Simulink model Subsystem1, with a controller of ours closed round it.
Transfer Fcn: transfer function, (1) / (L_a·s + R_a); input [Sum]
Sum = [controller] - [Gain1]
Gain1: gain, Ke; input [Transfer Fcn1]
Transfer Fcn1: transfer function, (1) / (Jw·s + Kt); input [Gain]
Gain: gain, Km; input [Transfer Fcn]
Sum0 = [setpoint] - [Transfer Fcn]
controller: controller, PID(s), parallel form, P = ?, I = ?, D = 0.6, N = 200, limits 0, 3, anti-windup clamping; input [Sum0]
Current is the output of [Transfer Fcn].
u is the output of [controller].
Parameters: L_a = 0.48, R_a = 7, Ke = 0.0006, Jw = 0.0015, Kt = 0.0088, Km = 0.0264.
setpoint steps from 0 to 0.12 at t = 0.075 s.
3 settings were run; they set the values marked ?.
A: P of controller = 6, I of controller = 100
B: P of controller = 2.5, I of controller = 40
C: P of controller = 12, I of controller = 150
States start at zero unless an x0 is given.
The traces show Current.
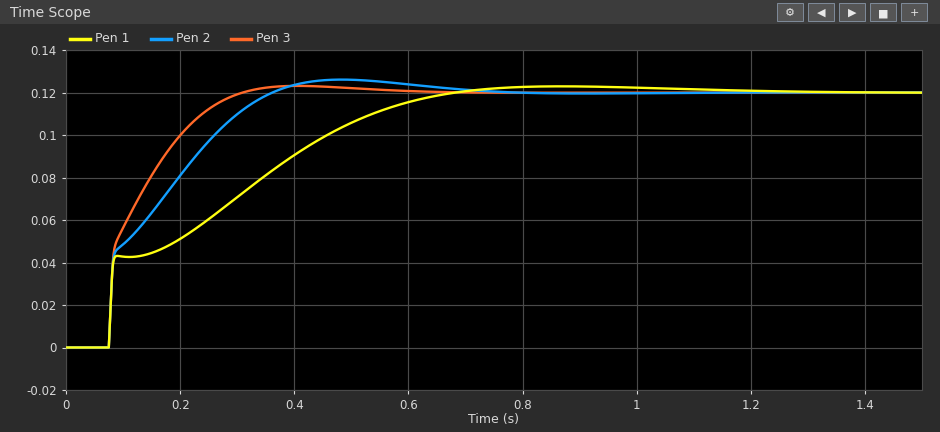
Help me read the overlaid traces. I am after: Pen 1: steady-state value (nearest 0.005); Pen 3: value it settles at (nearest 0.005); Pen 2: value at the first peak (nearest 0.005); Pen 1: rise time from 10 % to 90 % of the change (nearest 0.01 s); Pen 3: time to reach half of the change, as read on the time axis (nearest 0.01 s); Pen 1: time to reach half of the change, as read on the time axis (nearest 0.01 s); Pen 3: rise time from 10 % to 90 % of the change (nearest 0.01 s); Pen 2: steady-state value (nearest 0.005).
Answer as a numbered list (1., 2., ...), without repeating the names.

1. 0.120
2. 0.120
3. 0.125
4. 0.44 s
5. 0.11 s
6. 0.25 s
7. 0.15 s
8. 0.120
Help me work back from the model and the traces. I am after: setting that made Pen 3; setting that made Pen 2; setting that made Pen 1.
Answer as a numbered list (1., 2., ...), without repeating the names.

1. C
2. A
3. B
